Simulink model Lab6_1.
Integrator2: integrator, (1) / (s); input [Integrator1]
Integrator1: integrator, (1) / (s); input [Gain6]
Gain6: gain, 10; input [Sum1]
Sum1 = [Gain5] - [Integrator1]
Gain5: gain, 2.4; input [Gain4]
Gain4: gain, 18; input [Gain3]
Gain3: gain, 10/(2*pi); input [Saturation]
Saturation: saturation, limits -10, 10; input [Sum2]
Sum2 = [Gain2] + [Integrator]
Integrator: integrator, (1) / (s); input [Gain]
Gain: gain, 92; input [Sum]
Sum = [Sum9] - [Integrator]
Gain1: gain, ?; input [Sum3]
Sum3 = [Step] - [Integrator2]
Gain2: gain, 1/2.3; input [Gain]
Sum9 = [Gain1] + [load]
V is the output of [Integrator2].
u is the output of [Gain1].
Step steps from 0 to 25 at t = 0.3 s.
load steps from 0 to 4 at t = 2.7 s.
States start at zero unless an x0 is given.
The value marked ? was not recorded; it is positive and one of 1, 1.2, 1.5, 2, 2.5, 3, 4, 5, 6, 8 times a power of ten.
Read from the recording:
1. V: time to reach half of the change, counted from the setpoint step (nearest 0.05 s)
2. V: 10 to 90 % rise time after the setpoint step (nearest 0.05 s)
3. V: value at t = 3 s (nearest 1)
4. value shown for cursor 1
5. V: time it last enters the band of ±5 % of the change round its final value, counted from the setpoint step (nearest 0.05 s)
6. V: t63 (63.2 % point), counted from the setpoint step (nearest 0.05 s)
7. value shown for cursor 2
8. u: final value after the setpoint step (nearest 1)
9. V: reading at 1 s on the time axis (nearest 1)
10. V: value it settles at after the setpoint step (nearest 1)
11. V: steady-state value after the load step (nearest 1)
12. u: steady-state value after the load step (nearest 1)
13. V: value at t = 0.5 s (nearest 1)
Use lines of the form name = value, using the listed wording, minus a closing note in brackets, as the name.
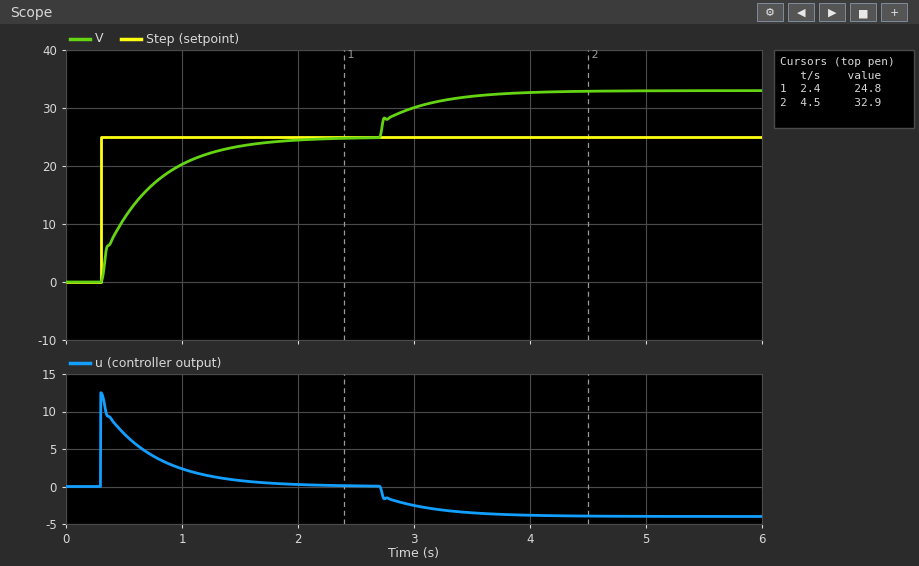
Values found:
V: time to reach half of the change, counted from the setpoint step = 0.25 s
V: 10 to 90 % rise time after the setpoint step = 0.95 s
V: value at t = 3 s = 30
value shown for cursor 1 = 24.8
V: time it last enters the band of ±5 % of the change round its final value, counted from the setpoint step = 1.30 s
V: t63 (63.2 % point), counted from the setpoint step = 0.40 s
value shown for cursor 2 = 32.9
u: final value after the setpoint step = 0
V: reading at 1 s on the time axis = 20
V: value it settles at after the setpoint step = 25
V: steady-state value after the load step = 33
u: steady-state value after the load step = -4
V: value at t = 0.5 s = 11
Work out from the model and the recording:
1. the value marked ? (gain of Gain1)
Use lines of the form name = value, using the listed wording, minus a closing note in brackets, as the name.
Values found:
the value marked ? = 0.5
